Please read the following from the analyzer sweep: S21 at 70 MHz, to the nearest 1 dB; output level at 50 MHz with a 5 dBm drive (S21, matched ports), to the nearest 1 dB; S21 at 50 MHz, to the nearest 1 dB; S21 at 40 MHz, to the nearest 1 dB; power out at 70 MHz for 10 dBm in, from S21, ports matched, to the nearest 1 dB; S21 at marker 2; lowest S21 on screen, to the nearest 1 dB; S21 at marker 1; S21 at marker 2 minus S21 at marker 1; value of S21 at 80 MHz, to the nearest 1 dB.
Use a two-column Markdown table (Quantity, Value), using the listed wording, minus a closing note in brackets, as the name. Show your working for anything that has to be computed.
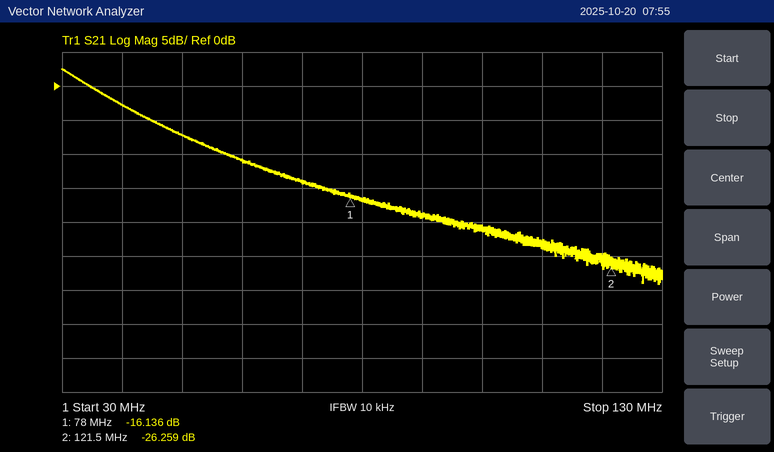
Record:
| Quantity | Value |
|---|---|
| S21 at 70 MHz, to the nearest 1 dB | -14 dB |
| output level at 50 MHz with a 5 dBm drive (S21, matched ports), to the nearest 1 dB | 5 dBm + (-7 dB) = -2 dBm |
| S21 at 50 MHz, to the nearest 1 dB | -7 dB |
| S21 at 40 MHz, to the nearest 1 dB | -3 dB |
| power out at 70 MHz for 10 dBm in, from S21, ports matched, to the nearest 1 dB | 10 dBm + (-14 dB) = -4 dBm |
| S21 at marker 2 | -26.259 dB |
| lowest S21 on screen, to the nearest 1 dB | -29 dB |
| S21 at marker 1 | -16.136 dB |
| S21 at marker 2 minus S21 at marker 1 | -26.259 − (-16.136) = -10.123 dB |
| value of S21 at 80 MHz, to the nearest 1 dB | -17 dB |
